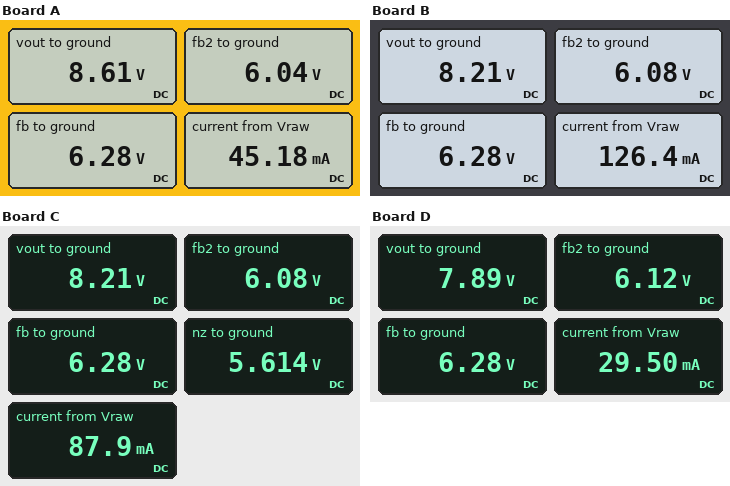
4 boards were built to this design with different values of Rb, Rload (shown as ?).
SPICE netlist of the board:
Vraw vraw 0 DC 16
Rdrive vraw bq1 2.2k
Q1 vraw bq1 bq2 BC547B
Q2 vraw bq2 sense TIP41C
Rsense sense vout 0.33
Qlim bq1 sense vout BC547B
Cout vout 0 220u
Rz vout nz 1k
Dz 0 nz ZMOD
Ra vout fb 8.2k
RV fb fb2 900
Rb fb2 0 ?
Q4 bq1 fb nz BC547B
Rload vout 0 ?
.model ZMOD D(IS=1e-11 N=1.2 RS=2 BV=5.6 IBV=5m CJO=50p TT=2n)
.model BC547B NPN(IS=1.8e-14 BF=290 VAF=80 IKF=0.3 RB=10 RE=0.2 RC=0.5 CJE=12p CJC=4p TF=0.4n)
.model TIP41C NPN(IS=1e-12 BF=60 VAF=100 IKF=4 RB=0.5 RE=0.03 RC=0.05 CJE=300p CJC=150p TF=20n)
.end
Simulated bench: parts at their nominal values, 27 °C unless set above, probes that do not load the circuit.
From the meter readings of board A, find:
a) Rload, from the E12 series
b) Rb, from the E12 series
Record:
220 Ω
22 kΩ
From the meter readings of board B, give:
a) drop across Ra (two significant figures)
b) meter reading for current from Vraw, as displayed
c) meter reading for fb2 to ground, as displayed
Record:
1.9 V
126.4 mA
6.08 V
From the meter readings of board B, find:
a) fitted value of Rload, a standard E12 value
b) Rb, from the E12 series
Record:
68 Ω
27 kΩ
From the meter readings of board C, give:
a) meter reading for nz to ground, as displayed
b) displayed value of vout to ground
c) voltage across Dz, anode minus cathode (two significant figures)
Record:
5.614 V
8.21 V
-5.6 V
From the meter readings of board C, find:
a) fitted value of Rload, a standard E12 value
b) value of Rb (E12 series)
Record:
100 Ω
27 kΩ
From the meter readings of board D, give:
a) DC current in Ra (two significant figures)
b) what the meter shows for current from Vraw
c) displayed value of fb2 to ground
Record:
200 µA
29.50 mA
6.12 V
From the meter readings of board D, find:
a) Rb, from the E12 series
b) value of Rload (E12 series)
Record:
33 kΩ
330 Ω
